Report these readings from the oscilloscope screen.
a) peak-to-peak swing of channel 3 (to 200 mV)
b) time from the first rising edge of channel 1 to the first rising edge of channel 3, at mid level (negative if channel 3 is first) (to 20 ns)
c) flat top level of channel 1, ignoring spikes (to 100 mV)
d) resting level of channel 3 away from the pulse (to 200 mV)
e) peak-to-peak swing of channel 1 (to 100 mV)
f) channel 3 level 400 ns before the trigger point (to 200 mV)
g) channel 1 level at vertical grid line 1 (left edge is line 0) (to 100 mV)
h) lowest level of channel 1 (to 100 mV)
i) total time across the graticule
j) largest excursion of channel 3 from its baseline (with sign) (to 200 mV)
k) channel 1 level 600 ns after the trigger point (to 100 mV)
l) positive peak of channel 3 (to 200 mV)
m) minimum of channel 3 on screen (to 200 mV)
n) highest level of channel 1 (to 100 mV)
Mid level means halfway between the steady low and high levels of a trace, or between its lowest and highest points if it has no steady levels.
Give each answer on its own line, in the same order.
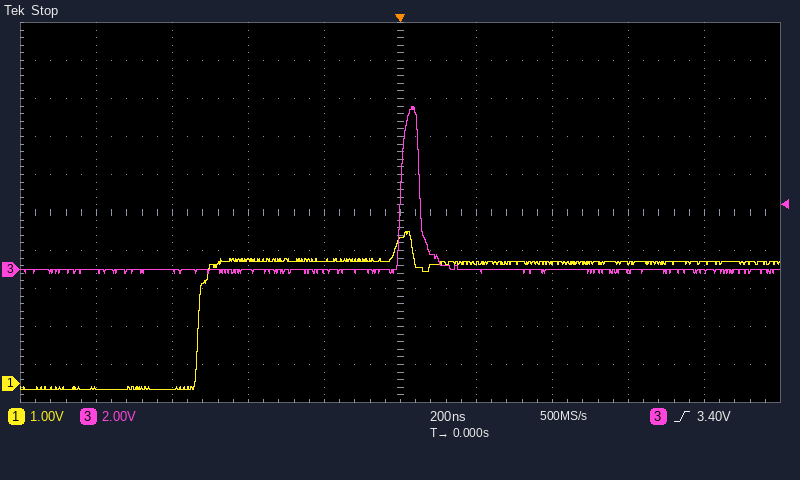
8.8 V
+540 ns
3.2 V
0.0 V
4.2 V
0.0 V
-100 mV
-200 mV
2 µs
+8.6 V
3.2 V
8.6 V
-200 mV
4.0 V
